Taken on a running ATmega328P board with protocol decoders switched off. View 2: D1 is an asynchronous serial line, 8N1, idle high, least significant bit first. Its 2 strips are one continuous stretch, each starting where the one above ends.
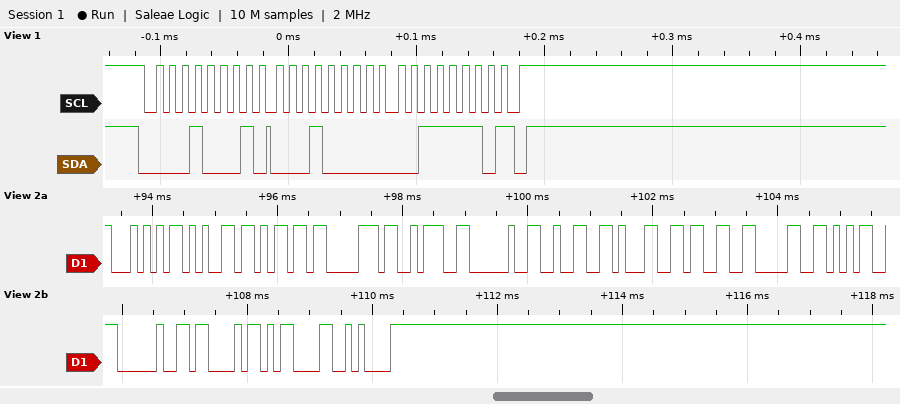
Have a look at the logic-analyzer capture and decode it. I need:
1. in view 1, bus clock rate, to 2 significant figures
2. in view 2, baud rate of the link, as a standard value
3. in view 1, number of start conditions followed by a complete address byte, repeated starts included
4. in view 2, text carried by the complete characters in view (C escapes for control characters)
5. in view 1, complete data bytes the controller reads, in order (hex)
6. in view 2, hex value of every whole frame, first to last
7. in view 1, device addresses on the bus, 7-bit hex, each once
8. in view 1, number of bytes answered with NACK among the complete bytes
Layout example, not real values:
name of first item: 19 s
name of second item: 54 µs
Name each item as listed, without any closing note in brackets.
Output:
in view 1, bus clock rate, to 2 significant figures: 100 kHz
in view 2, baud rate of the link, as a standard value: 9600 baud
in view 1, number of start conditions followed by a complete address byte, repeated starts included: 1
in view 2, text carried by the complete characters in view: "Temp: 21305 C\r\n"
in view 1, complete data bytes the controller reads, in order: 10 3E
in view 2, hex value of every whole frame, first to last: 0x54 0x65 0x6D 0x70 0x3A 0x20 0x32 0x31 0x33 0x30 0x35 0x20 0x43 0x0D 0x0A
in view 1, device addresses on the bus, 7-bit hex, each once: 0x08
in view 1, number of bytes answered with NACK among the complete bytes: 1
